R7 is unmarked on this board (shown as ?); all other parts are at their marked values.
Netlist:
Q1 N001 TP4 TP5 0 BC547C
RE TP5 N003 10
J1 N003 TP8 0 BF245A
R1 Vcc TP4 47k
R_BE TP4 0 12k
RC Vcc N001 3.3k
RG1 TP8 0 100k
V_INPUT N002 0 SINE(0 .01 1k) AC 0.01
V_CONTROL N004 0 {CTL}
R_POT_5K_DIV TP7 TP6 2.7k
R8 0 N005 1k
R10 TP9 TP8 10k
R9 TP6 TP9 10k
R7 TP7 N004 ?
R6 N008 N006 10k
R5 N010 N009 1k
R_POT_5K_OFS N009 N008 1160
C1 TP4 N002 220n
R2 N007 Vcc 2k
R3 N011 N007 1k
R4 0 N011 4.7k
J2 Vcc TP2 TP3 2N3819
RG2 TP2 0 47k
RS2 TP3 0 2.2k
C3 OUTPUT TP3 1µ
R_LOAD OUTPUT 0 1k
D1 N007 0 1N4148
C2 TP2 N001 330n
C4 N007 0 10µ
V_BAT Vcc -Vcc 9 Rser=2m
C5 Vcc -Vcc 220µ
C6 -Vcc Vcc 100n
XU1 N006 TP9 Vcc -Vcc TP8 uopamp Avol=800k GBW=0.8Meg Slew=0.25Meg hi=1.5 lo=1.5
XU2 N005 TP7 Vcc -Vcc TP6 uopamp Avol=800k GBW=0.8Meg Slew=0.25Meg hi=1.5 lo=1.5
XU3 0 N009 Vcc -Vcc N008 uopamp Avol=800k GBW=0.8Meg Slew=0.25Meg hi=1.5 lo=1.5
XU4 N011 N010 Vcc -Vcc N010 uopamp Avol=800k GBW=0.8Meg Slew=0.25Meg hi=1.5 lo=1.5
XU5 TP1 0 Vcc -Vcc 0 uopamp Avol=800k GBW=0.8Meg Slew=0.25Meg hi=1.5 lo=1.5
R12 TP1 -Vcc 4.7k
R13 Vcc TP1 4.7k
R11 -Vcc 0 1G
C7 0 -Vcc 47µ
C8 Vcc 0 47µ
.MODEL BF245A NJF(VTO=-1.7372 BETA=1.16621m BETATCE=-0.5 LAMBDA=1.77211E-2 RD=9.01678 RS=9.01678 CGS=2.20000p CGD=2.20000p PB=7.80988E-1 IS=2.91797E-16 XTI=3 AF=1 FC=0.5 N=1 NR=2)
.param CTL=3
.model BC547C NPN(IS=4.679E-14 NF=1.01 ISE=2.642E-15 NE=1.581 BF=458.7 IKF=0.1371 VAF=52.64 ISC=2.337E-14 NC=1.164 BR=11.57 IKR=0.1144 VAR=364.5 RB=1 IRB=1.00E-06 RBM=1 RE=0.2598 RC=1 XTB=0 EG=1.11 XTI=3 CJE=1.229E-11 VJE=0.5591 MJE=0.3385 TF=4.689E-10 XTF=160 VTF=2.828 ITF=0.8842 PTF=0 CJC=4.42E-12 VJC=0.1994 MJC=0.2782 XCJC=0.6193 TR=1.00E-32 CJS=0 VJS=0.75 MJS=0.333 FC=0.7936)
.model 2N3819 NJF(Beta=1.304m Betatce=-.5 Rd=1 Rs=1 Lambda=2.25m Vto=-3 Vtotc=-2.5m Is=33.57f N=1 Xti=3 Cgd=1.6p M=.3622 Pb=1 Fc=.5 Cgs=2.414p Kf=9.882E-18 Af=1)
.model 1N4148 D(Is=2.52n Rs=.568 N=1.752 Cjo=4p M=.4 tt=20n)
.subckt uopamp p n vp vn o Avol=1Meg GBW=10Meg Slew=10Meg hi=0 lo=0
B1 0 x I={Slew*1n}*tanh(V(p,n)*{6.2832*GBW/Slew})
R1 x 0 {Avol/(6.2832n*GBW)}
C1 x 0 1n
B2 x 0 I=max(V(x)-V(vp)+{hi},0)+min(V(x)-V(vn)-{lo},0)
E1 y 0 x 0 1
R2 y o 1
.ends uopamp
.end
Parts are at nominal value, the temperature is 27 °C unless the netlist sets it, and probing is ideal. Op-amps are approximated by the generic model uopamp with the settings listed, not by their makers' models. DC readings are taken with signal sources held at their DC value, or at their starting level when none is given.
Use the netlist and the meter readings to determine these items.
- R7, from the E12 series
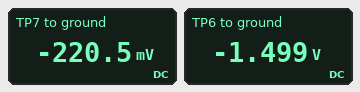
6.8 kΩ
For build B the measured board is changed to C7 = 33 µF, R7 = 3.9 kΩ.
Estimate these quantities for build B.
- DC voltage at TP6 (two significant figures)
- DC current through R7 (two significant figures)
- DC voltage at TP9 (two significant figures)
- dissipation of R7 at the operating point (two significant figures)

-2.1 V
770 µA
-1.8 V
2.3 mW
